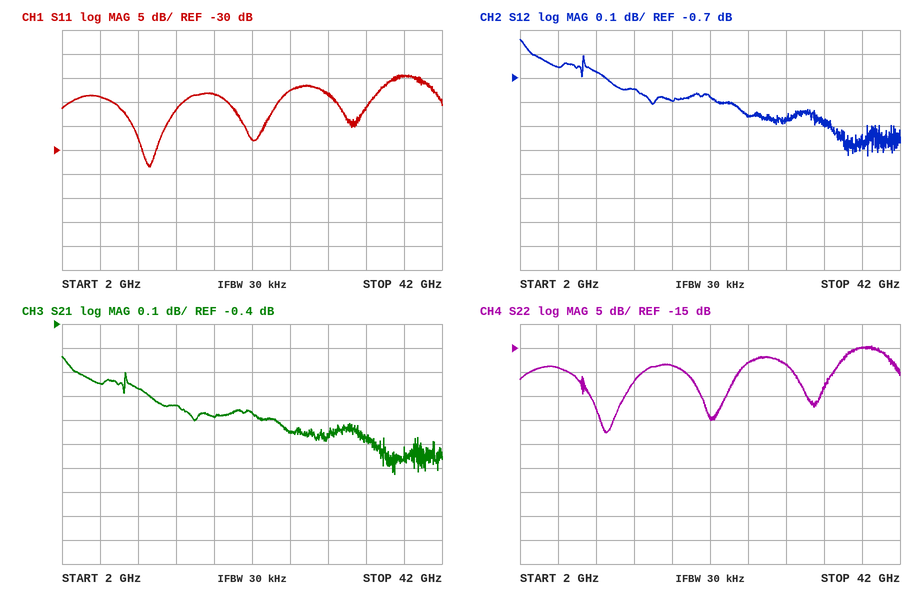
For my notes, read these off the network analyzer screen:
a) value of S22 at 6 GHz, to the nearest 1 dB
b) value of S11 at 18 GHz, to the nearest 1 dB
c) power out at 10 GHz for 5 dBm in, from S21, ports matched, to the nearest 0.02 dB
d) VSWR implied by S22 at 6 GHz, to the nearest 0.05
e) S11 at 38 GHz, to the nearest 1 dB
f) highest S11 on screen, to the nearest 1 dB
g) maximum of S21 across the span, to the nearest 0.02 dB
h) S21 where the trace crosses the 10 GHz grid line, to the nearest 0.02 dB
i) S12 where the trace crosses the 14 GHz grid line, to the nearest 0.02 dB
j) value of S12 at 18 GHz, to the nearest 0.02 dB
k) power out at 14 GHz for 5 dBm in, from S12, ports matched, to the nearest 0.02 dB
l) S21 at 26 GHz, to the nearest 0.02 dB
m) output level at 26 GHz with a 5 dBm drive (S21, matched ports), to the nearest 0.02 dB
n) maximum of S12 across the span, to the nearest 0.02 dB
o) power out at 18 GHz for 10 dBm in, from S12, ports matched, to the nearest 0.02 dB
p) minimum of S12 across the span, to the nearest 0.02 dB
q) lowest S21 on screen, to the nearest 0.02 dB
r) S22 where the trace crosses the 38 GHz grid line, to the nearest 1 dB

-19 dB
-18 dB
4.34 dBm
1.25
-15 dB
-14 dB
-0.54 dB
-0.66 dB
-0.74 dB
-0.80 dB
4.26 dBm
-0.84 dB
4.16 dBm
-0.54 dB
9.20 dBm
-1.02 dB
-1.02 dB
-15 dB
